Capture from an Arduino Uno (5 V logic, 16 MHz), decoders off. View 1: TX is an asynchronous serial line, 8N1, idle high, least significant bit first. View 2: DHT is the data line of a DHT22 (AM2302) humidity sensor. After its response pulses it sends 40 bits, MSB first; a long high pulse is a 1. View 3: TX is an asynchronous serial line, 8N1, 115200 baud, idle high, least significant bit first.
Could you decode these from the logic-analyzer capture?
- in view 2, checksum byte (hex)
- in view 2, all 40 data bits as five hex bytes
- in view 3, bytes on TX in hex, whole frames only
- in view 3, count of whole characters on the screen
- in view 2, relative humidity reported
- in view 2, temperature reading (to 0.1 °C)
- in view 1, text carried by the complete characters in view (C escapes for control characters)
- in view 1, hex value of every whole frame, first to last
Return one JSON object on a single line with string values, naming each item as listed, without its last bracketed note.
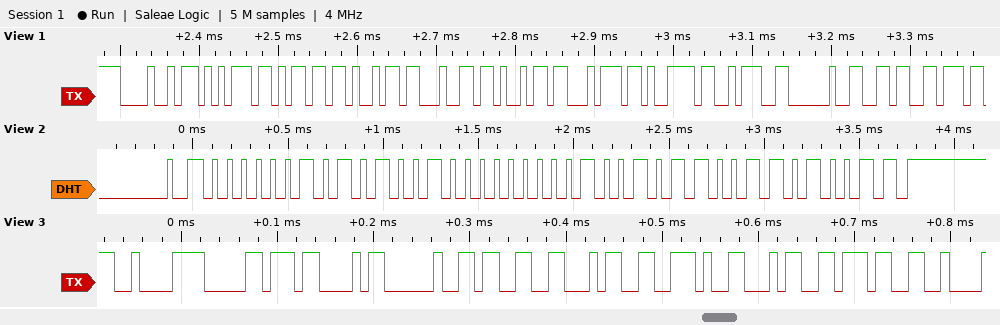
{"in view 2, checksum byte": "0xD3", "in view 2, all 40 data bits as five hex bytes": "02 A4 01 2C D3", "in view 3, bytes on TX in hex, whole frames only": "C2 B0 43 20 33 34 2E 34 37", "in view 3, count of whole characters on the screen": "9", "in view 2, relative humidity reported": "67.6 %", "in view 2, temperature reading": "30.0 °C", "in view 1, text carried by the complete characters in view": "\"Humidity: 6\"", "in view 1, hex value of every whole frame, first to last": "48 75 6D 69 64 69 74 79 3A 20 36"}
